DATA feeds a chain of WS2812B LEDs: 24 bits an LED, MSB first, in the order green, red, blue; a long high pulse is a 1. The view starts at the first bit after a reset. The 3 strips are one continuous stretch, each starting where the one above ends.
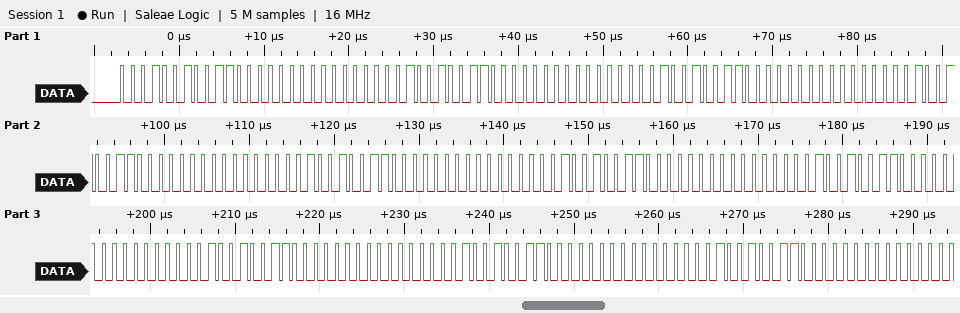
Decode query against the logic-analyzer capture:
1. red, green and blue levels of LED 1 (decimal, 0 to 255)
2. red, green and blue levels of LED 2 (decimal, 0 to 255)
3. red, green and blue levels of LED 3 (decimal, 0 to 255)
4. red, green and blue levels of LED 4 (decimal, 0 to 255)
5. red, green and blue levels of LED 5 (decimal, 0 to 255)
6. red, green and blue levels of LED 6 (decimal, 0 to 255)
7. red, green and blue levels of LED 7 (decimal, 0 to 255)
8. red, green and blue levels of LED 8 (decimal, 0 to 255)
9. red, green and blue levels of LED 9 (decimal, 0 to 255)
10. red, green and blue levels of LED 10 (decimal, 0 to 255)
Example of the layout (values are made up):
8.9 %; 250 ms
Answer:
96, 18, 0; 96, 18, 0; 96, 18, 0; 96, 18, 0; 96, 18, 0; 96, 18, 0; 96, 18, 0; 96, 18, 0; 96, 18, 0; 96, 18, 0
